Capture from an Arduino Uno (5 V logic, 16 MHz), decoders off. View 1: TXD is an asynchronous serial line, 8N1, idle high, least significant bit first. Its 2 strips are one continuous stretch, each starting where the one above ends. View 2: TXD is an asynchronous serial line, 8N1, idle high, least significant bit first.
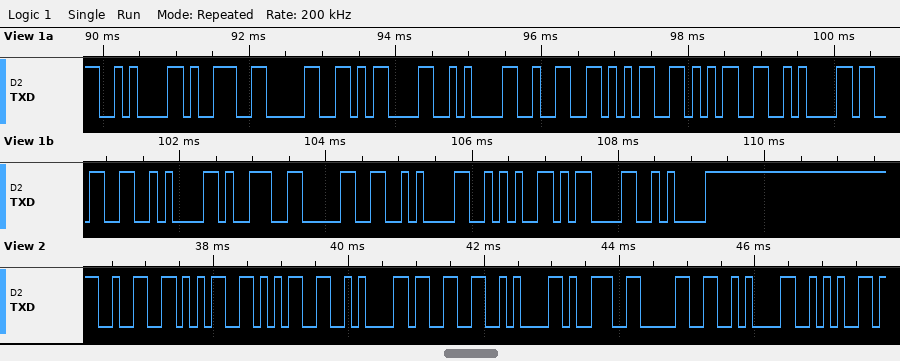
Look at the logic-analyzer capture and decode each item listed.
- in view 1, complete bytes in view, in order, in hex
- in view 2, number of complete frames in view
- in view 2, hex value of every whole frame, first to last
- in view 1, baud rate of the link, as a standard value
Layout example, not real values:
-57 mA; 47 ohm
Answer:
0x0A 0x39 0x30 0x0D 0x0A 0x32 0x35 0x35 0x0A 0x33 0x0A 0x39 0x30 0x0A 0x2A 0x0D 0x0A; 10; 32 35 35 0A 33 0A 39 30 0A 2A; 9600 baud
